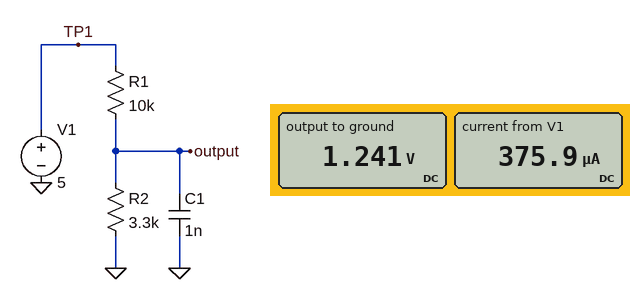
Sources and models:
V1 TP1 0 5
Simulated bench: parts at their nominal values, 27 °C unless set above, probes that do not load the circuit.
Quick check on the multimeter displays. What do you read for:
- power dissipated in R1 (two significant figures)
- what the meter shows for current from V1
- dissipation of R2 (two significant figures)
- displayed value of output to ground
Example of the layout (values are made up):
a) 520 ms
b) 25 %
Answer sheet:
a) 1.4 mW
b) 375.9 µA
c) 470 µW
d) 1.241 V
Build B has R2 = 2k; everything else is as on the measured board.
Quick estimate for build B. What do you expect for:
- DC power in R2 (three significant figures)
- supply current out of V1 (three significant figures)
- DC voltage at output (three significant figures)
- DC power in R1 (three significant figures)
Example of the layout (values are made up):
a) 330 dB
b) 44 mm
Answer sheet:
a) 347 µW
b) 417 µA
c) 833 mV
d) 1.74 mW
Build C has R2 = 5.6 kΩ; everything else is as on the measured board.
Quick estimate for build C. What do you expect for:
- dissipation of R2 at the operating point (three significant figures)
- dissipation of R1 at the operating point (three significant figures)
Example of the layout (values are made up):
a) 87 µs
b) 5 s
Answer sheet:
a) 575 µW
b) 1.03 mW
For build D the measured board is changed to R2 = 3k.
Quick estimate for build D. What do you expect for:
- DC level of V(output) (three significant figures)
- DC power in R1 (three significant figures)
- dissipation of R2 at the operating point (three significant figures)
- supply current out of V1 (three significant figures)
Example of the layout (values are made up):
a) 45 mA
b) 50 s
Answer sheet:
a) 1.15 V
b) 1.48 mW
c) 444 µW
d) 385 µA
